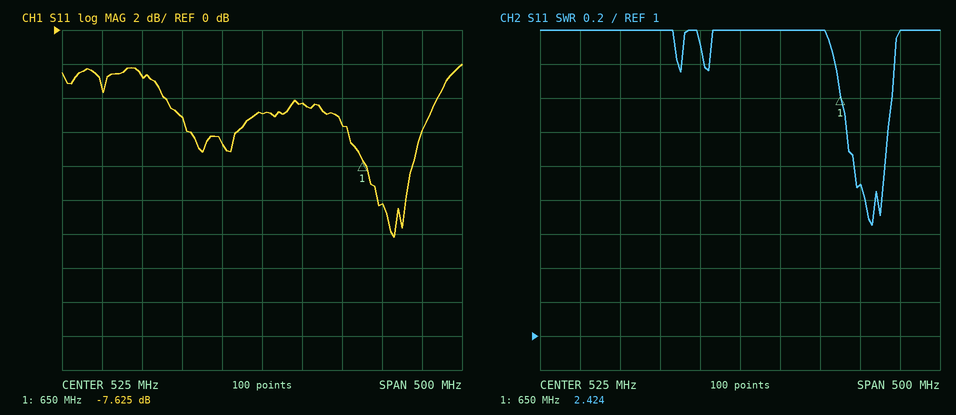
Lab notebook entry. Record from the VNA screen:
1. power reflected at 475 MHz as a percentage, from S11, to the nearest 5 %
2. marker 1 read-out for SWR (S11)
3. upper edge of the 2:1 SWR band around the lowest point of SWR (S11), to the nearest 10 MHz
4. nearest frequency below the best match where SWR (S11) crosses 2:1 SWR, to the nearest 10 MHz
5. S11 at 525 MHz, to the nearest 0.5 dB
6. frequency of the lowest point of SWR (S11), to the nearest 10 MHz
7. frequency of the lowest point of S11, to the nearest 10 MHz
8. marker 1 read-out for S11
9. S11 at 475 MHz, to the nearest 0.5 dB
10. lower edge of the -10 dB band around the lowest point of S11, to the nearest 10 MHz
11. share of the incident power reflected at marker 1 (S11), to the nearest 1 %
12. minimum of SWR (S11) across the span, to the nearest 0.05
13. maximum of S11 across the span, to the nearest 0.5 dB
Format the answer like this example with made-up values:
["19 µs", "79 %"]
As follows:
["20 %", "2.424", "710 MHz", "670 MHz", "-5.0 dB", "690 MHz", "690 MHz", "-7.625 dB", "-6.5 dB", "670 MHz", "17 %", "1.65", "-2.0 dB"]
